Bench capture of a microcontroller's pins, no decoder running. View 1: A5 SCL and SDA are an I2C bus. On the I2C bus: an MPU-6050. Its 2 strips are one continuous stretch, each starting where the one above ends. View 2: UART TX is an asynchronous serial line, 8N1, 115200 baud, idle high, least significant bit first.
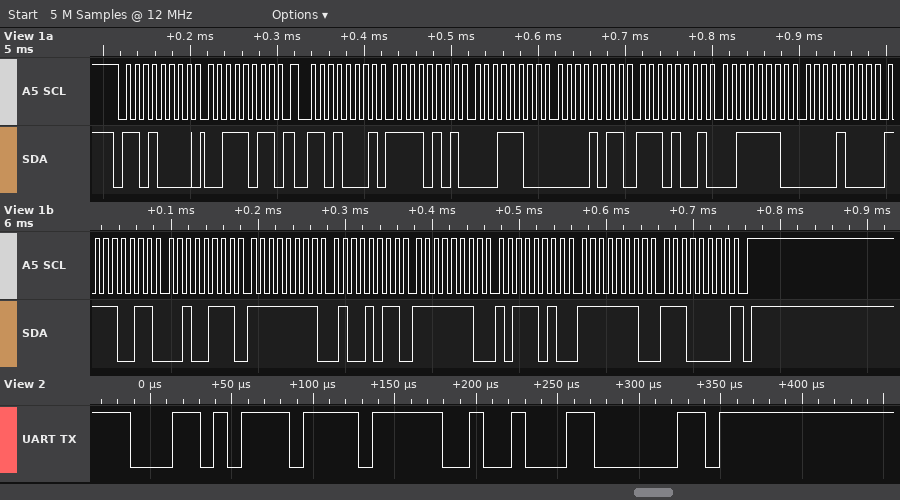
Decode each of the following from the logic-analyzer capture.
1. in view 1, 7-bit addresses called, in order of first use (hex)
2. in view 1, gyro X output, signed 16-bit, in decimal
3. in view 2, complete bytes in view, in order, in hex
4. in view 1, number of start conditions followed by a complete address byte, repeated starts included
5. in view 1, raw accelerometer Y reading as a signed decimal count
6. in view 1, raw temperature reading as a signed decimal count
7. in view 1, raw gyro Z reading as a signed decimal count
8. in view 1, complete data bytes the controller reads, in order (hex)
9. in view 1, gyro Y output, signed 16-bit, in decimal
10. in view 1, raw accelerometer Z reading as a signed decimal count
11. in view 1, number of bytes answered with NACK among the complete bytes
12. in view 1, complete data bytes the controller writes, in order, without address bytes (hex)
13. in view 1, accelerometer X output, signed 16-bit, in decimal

0x68
-181
AC EF 12 60
2
3049
-3289
-288
F5 1C 0B E9 3E 08 F3 27 FF 4B FE BA FE E0
-326
15880
1
3B
-2788
